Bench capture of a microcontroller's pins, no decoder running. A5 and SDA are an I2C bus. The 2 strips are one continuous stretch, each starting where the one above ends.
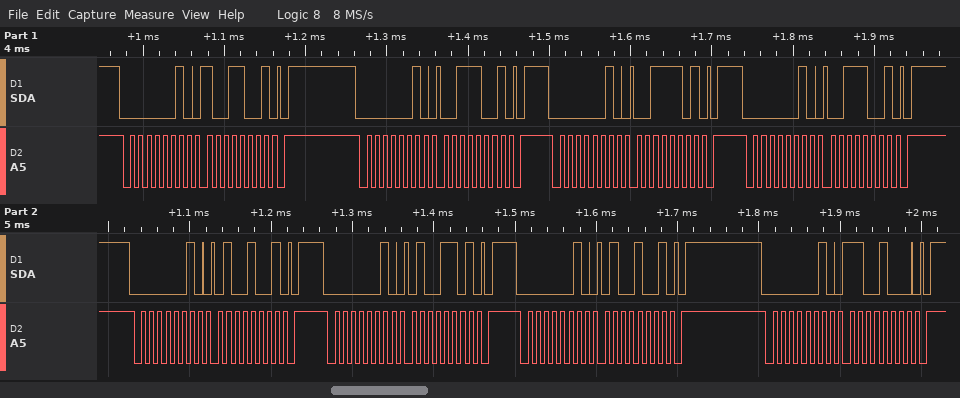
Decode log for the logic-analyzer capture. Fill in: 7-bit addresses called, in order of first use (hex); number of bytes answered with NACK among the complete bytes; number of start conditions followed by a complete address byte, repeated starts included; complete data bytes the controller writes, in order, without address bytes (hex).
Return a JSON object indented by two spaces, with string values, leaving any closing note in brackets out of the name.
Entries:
{
  "7-bit addresses called, in order of first use": "0x01",
  "number of bytes answered with NACK among the complete bytes": "0",
  "number of start conditions followed by a complete address byte, repeated starts included": "8",
  "complete data bytes the controller writes, in order, without address bytes": "99 39 3D 39 49 4D 49 C8"
}
